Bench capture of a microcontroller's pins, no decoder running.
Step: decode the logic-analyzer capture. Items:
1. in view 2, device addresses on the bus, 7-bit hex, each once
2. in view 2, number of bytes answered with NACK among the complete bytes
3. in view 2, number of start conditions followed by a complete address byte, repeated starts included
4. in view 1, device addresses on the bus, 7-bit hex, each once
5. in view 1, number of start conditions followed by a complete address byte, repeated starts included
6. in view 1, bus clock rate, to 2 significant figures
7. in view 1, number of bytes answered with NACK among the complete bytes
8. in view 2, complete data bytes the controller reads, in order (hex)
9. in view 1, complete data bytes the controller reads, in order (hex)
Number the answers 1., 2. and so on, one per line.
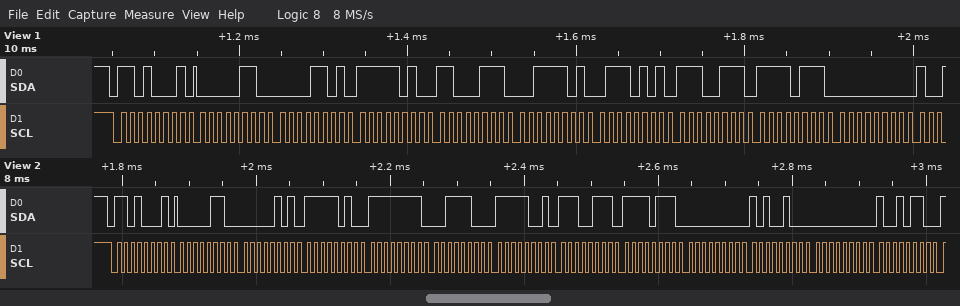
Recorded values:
1. 0x68
2. 0
3. 1
4. 0x68
5. 1
6. 100 kHz
7. 0
8. 06 05 FA FF 3C F9 E7 F7 00 A4 00 96
9. 06 0D FA C7 3D 75 E7 F7 00
